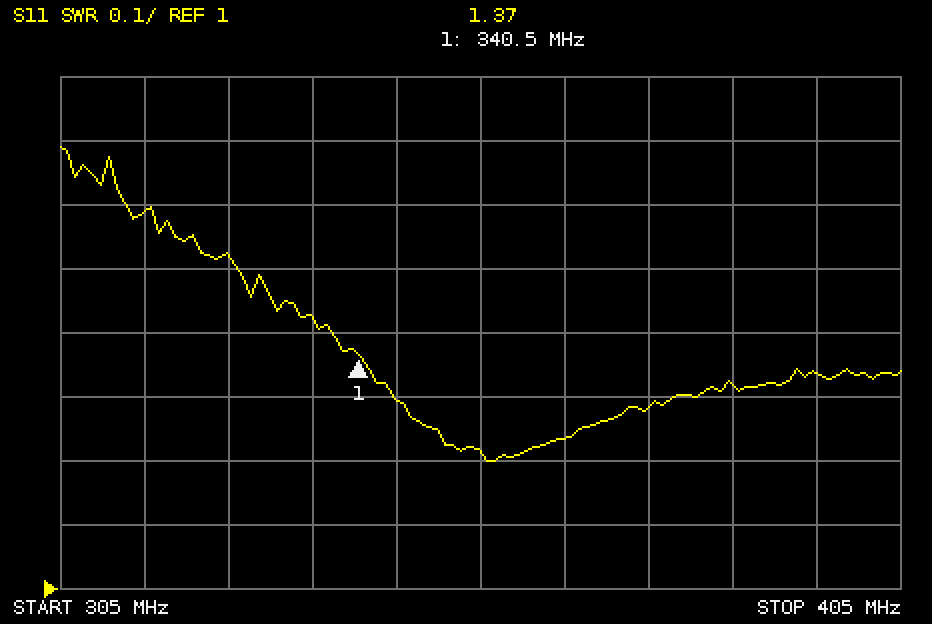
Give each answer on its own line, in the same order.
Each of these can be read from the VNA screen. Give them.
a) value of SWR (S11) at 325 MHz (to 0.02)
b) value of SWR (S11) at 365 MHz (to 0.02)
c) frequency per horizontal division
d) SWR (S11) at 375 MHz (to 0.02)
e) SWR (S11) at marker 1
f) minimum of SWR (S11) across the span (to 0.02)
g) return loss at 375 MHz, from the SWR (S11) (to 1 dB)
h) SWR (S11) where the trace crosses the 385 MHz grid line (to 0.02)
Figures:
1.52
1.24
10 MHz
1.28
1.37
1.20
18 dB
1.32
